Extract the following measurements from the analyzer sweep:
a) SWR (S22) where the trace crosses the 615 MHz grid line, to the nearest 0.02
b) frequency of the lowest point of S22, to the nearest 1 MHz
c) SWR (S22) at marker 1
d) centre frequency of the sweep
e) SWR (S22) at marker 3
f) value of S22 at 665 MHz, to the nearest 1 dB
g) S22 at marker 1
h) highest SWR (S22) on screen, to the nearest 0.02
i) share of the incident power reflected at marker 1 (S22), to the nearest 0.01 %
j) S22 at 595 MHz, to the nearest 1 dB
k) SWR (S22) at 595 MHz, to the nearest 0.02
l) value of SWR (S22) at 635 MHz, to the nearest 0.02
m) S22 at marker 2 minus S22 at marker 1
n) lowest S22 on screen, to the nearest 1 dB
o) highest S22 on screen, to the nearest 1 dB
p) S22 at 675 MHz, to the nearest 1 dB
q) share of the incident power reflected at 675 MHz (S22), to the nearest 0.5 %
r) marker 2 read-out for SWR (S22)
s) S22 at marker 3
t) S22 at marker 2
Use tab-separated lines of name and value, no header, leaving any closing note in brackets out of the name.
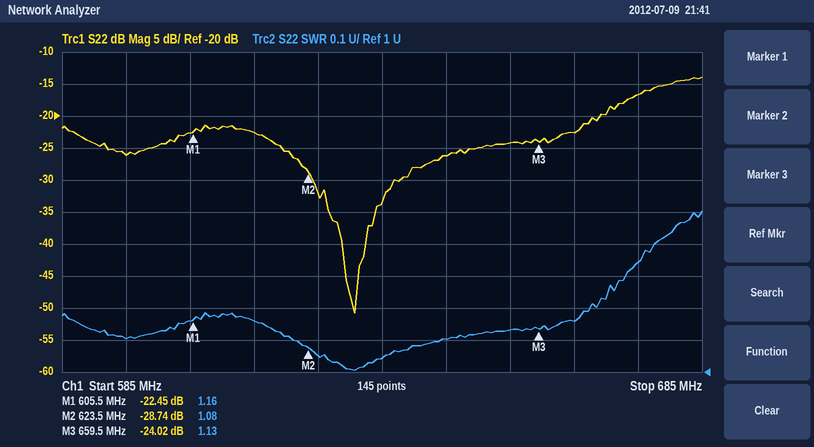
SWR (S22) where the trace crosses the 615 MHz grid line, to the nearest 0.02	1.16
frequency of the lowest point of S22, to the nearest 1 MHz	631 MHz
SWR (S22) at marker 1	1.16
centre frequency of the sweep	635 MHz
SWR (S22) at marker 3	1.13
value of S22 at 665 MHz, to the nearest 1 dB	-23 dB
S22 at marker 1	-22.45 dB
highest SWR (S22) on screen, to the nearest 0.02	1.50
share of the incident power reflected at marker 1 (S22), to the nearest 0.01 %	0.57 %
S22 at 595 MHz, to the nearest 1 dB	-26 dB
SWR (S22) at 595 MHz, to the nearest 0.02	1.10
value of SWR (S22) at 635 MHz, to the nearest 0.02	1.04
S22 at marker 2 minus S22 at marker 1	-6.29 dB
lowest S22 on screen, to the nearest 1 dB	-51 dB
highest S22 on screen, to the nearest 1 dB	-14 dB
S22 at 675 MHz, to the nearest 1 dB	-17 dB
share of the incident power reflected at 675 MHz (S22), to the nearest 0.5 %	2.0 %
marker 2 read-out for SWR	1.08
S22 at marker 3	-24.02 dB
S22 at marker 2	-28.74 dB
